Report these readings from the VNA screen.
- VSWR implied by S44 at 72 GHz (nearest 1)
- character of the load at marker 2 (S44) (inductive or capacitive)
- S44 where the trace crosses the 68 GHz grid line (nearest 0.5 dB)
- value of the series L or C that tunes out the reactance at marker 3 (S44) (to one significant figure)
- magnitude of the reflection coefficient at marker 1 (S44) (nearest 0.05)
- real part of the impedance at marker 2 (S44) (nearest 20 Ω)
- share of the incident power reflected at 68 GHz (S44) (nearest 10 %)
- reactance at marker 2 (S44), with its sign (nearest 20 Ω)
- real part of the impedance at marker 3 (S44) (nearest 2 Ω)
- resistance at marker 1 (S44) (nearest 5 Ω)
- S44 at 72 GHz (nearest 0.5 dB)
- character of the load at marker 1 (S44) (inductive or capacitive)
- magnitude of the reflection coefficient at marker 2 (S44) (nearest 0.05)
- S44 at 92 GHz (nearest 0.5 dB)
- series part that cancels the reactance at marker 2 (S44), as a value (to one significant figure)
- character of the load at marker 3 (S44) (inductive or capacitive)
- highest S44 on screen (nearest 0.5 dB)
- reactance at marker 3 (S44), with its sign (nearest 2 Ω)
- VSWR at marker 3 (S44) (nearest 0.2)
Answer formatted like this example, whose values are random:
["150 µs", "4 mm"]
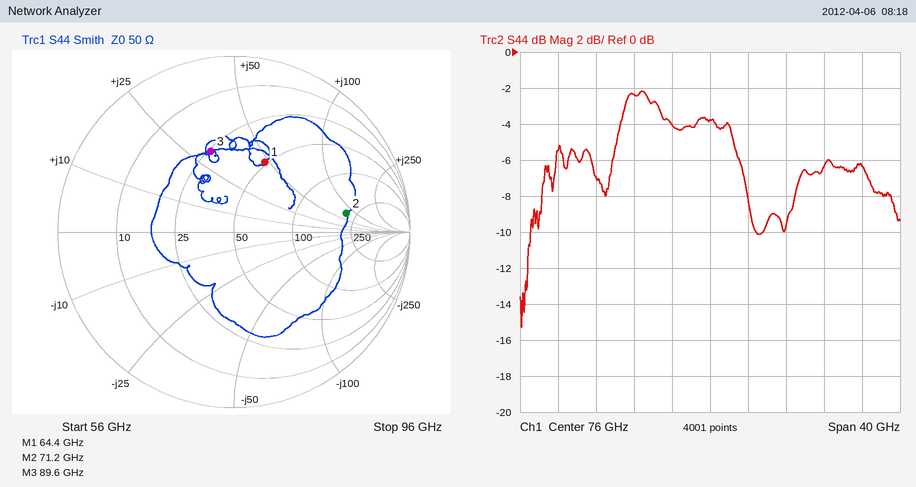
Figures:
["4", "inductive", "-2.5 dB", "60 fF", "0.45", "200 Ω", "60 %", "+80 Ω", "26 Ω", "50 Ω", "-4.0 dB", "inductive", "0.65", "-6.5 dB", "30 fF", "inductive", "-2.0 dB", "+30 Ω", "2.8"]
